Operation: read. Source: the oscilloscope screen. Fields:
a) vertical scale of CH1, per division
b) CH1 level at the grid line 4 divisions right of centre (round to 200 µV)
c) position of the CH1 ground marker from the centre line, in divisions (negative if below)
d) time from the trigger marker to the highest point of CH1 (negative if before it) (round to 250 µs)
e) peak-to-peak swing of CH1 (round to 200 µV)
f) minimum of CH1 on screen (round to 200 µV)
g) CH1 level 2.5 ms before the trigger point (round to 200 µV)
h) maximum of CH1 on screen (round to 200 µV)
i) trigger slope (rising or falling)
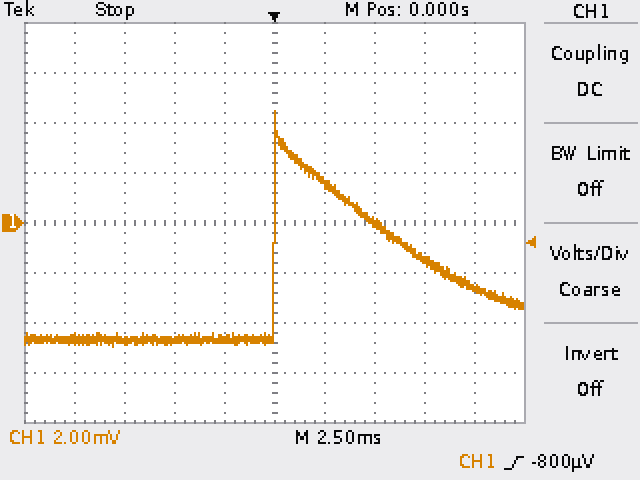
2 mV
-2.6 mV
0.0 div
0.00 ms
9.4 mV
-5.0 mV
-4.6 mV
4.4 mV
rising
